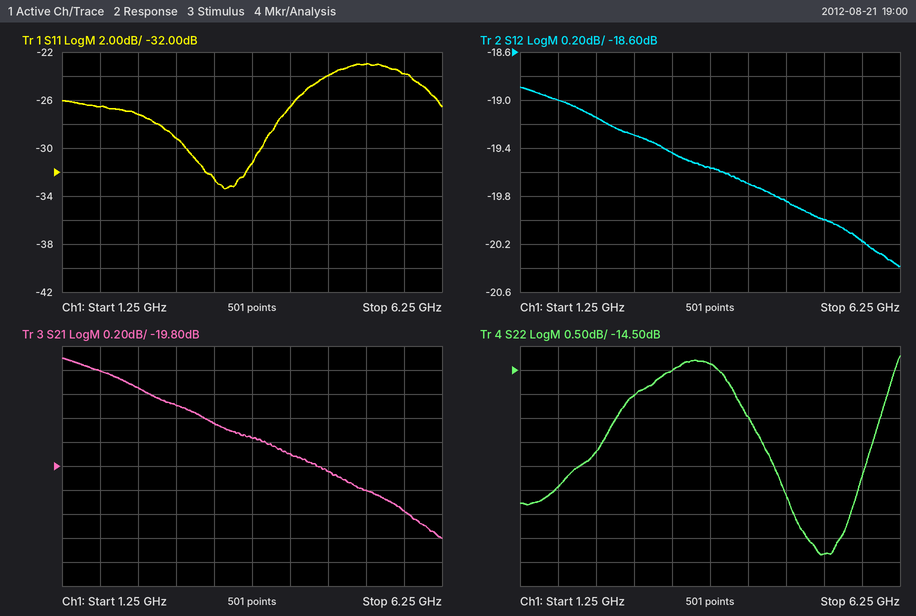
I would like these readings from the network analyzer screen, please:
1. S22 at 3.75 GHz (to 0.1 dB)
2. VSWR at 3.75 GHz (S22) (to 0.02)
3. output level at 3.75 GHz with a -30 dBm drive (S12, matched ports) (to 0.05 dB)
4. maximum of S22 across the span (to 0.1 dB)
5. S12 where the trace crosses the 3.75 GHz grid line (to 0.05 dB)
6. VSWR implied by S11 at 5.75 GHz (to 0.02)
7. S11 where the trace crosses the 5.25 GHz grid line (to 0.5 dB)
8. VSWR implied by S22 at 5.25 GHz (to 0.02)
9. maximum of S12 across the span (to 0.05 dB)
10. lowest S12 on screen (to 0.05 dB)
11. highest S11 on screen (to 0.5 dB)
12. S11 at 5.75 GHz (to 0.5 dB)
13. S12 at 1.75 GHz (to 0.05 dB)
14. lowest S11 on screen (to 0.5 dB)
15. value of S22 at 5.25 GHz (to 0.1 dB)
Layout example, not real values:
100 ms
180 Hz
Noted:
-14.4 dB
1.48
-49.55 dBm
-14.2 dB
-19.55 dB
1.14
-23.0 dB
1.28
-18.90 dB
-20.40 dB
-23.0 dB
-24.0 dB
-19.00 dB
-33.5 dB
-18.3 dB
